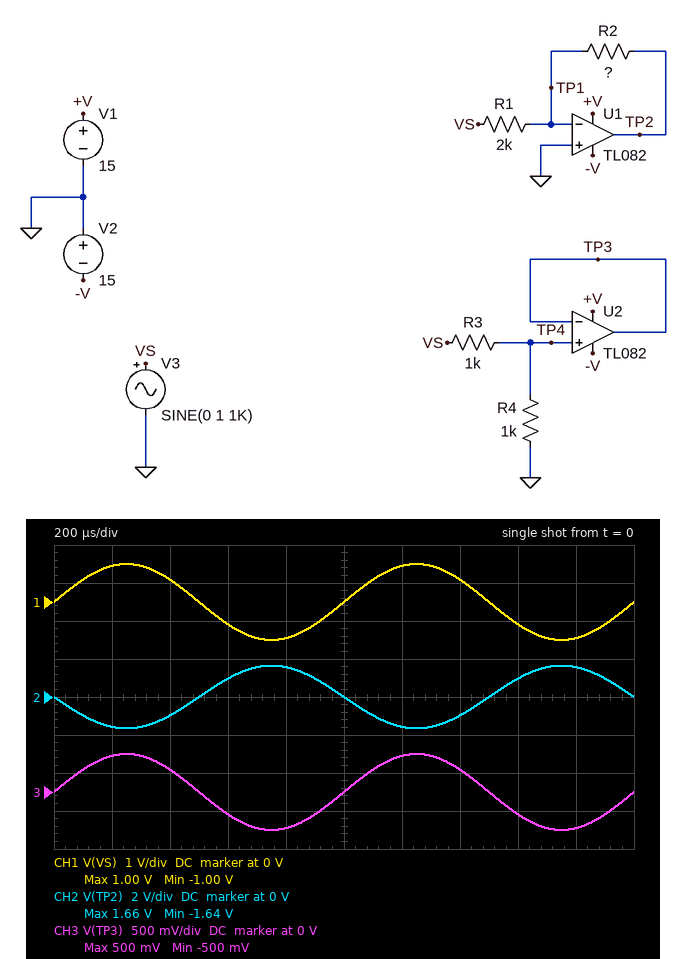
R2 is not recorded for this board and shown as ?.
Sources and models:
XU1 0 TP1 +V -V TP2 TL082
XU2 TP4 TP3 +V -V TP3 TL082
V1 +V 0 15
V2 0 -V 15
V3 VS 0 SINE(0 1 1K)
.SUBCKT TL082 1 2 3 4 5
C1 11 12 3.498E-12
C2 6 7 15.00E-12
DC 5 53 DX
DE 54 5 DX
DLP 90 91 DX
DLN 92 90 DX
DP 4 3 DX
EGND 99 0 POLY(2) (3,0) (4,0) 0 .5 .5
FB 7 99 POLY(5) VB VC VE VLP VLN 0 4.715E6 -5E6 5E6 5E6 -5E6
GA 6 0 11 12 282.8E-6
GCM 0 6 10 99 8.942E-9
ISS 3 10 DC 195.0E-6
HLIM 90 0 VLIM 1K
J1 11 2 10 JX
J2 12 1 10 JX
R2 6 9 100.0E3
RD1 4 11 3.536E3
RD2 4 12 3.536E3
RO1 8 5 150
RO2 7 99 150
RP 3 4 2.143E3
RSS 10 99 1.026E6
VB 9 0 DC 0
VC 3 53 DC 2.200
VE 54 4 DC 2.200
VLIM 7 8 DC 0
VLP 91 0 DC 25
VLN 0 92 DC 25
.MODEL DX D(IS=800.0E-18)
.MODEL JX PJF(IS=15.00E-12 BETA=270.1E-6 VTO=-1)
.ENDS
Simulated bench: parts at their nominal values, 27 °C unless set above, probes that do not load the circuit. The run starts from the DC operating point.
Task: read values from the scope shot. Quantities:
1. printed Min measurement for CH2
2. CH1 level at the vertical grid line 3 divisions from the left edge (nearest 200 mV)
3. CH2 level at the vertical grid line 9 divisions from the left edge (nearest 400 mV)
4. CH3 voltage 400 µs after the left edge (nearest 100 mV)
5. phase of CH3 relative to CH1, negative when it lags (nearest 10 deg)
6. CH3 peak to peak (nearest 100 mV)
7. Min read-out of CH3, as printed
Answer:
-1.64 V
-600 mV
1.6 V
300 mV
0 deg
1.0 V
-500 mV
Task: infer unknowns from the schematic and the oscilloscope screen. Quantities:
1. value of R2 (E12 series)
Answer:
3.3 kΩ
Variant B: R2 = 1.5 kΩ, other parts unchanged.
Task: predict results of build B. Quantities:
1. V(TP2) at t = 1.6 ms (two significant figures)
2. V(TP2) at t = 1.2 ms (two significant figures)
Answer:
440 mV
-710 mV
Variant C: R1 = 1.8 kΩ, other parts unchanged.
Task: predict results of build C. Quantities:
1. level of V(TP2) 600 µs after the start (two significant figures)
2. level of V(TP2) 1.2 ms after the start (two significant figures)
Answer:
1.1 V
-1.7 V
